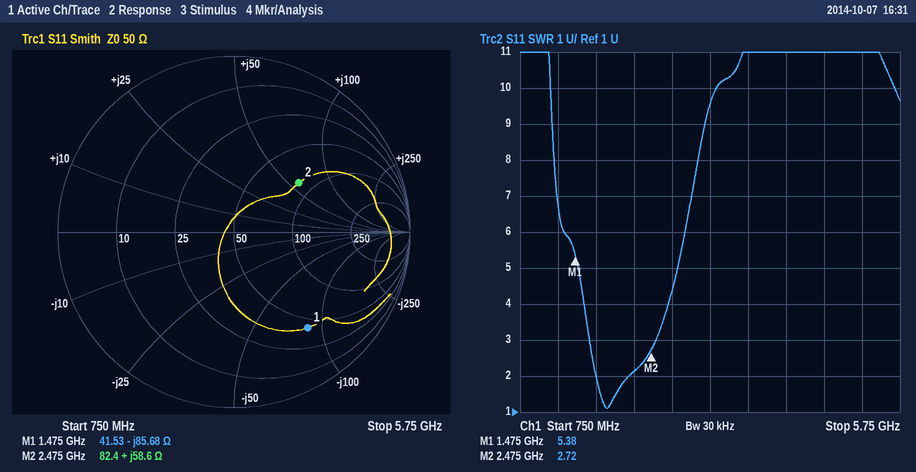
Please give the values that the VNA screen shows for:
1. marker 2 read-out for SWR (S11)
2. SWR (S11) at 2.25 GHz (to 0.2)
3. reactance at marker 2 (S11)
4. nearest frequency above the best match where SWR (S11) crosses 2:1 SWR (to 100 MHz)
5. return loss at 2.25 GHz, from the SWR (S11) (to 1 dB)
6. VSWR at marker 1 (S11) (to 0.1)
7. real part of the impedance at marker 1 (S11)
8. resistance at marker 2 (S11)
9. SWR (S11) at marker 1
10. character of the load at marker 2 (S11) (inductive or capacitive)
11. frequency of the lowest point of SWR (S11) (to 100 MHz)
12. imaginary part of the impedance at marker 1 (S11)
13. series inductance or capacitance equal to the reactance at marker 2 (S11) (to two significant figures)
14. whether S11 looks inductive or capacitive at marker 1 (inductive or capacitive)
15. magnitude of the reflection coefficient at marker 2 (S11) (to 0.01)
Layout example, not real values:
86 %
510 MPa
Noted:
2.72
2.2
+58.6 Ω
2.2 GHz
9 dB
5.4
41.53 Ω
82.4 Ω
5.38
inductive
1.9 GHz
-85.68 Ω
3.8 nH
capacitive
0.46
